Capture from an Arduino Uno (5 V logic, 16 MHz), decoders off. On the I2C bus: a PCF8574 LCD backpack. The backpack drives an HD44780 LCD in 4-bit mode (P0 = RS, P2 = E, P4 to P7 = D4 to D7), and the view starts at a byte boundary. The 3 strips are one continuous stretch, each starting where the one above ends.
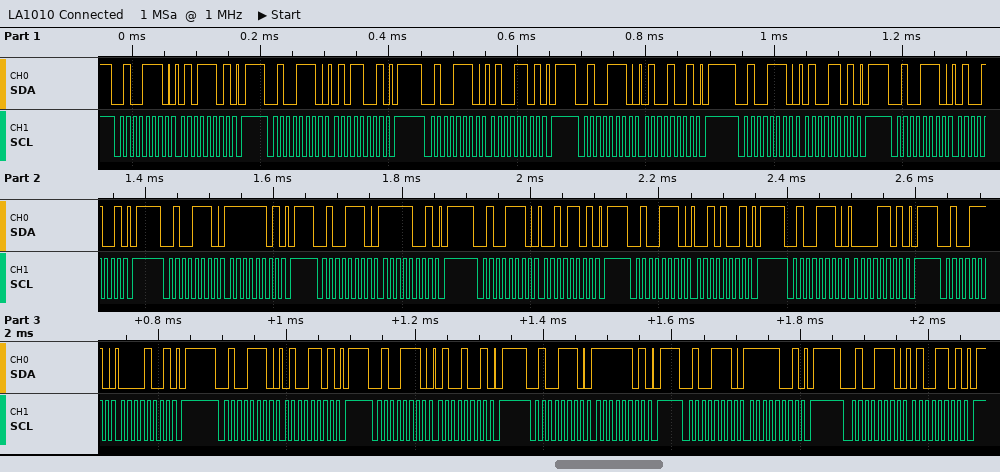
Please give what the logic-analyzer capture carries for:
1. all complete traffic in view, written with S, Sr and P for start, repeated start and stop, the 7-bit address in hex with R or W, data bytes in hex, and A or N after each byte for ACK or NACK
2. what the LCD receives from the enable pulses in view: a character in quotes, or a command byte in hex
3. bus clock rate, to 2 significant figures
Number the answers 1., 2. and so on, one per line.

1. S 27W A 5D A P S 27W A 59 A P S 27W A 4D A P S 27W A 49 A P S 27W A 4D A P S 27W A 49 A P S 27W A FD A P S 27W A F9 A P S 27W A 2D A P S 27W A 29 A P S 27W A 0D A P S 27W A 09 A P S 27W A 4D A P S 27W A 49 A P S 27W A FD A P S 27W A F9 A P S 27W A 4D A P
2. 'T' 'O' ' ' 'O'
3. 100 kHz
